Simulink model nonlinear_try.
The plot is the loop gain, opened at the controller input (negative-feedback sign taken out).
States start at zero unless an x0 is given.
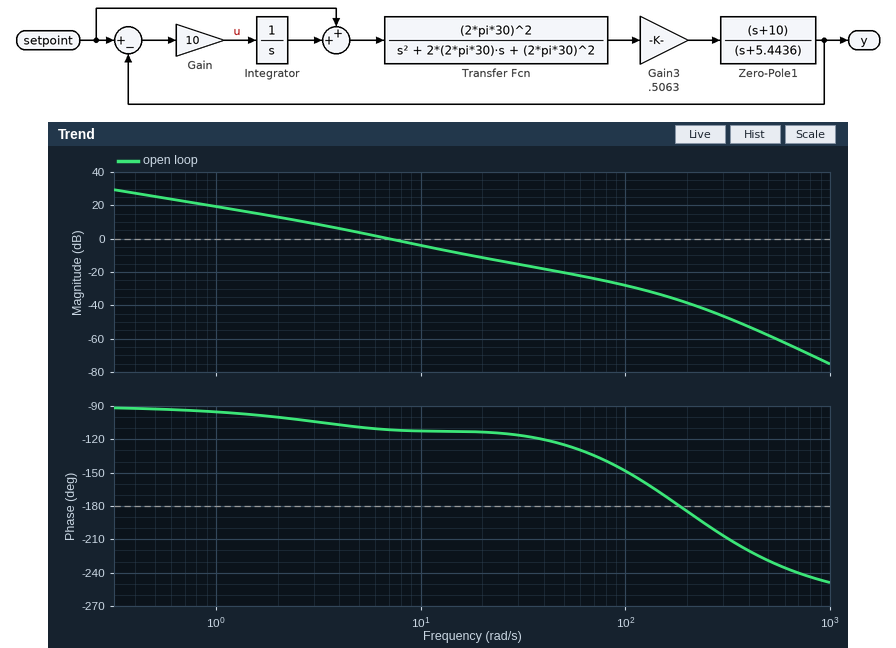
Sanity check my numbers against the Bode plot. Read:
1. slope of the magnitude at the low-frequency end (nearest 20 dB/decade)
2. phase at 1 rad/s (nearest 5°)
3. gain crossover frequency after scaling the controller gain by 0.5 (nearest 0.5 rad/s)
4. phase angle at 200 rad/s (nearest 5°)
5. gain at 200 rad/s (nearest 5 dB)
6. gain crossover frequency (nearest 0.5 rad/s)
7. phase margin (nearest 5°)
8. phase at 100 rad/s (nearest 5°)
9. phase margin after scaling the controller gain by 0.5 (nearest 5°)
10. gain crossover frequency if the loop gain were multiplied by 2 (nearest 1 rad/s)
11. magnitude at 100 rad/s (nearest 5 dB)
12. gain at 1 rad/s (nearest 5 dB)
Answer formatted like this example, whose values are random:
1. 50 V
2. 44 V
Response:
1. -20 dB/decade
2. -95°
3. 4.0 rad/s
4. -185°
5. -40 dB
6. 7.0 rad/s
7. 70°
8. -150°
9. 75°
10. 12 rad/s
11. -30 dB
12. 20 dB
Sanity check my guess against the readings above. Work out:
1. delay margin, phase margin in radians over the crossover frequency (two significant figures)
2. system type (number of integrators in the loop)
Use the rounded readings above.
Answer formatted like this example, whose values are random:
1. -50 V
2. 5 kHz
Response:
1. 0.17 s
2. 1
